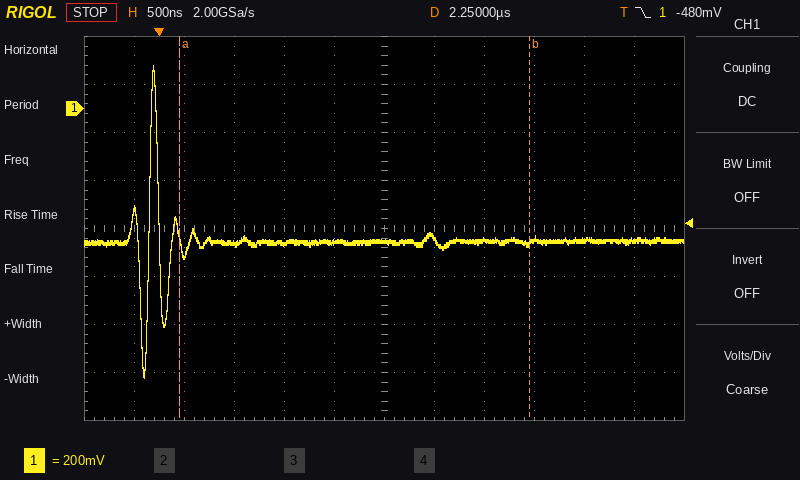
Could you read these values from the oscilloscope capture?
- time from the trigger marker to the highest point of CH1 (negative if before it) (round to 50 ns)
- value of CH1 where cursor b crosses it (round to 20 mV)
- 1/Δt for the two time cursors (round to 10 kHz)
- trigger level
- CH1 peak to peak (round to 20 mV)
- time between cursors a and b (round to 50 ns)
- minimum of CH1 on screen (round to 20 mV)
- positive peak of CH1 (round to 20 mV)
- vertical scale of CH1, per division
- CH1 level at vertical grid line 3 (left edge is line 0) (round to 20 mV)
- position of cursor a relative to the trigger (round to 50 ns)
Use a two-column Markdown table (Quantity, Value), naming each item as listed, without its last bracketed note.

| Quantity | Value |
|---|---|
| time from the trigger marker to the highest point of CH1 (negative if before it) | -50 ns |
| value of CH1 where cursor b crosses it | -560 mV |
| 1/Δt for the two time cursors | 290 kHz |
| trigger level | -480 mV |
| CH1 peak to peak | 1.30 V |
| time between cursors a and b | 3.50 µs |
| minimum of CH1 on screen | -1.12 V |
| positive peak of CH1 | 180 mV |
| vertical scale of CH1, per division | 200 mV |
| CH1 level at vertical grid line 3 (left edge is line 0) | -560 mV |
| position of cursor a relative to the trigger | +200 ns |
